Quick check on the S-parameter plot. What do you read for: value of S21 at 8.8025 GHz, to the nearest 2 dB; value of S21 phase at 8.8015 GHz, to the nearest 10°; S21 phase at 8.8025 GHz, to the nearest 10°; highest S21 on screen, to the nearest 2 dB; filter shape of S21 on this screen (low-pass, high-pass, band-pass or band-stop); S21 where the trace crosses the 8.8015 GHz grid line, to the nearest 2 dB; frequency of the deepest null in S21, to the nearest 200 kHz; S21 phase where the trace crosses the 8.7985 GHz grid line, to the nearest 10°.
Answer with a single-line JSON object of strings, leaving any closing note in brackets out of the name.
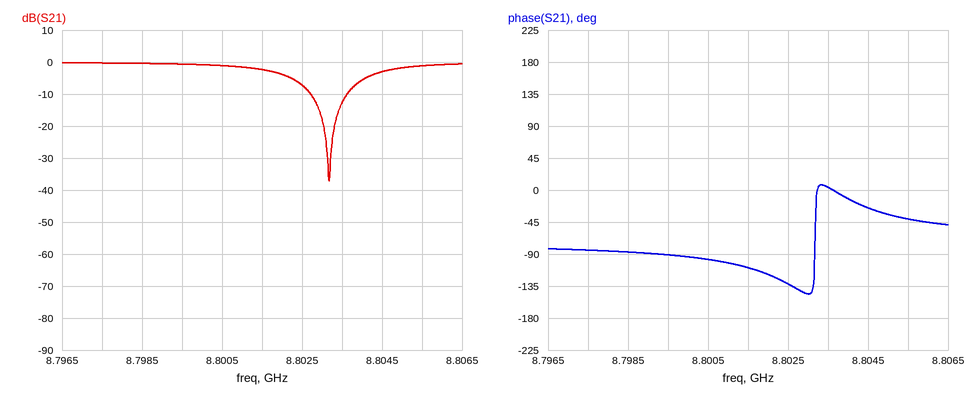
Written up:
{"value of S21 at 8.8025 GHz, to the nearest 2 dB": "-8 dB", "value of S21 phase at 8.8015 GHz, to the nearest 10°": "-110°", "S21 phase at 8.8025 GHz, to the nearest 10°": "-130°", "highest S21 on screen, to the nearest 2 dB": "0 dB", "filter shape of S21 on this screen": "band-stop", "S21 where the trace crosses the 8.8015 GHz grid line, to the nearest 2 dB": "-2 dB", "frequency of the deepest null in S21, to the nearest 200 kHz": "8.8032 GHz", "S21 phase where the trace crosses the 8.7985 GHz grid line, to the nearest 10°": "-90°"}
